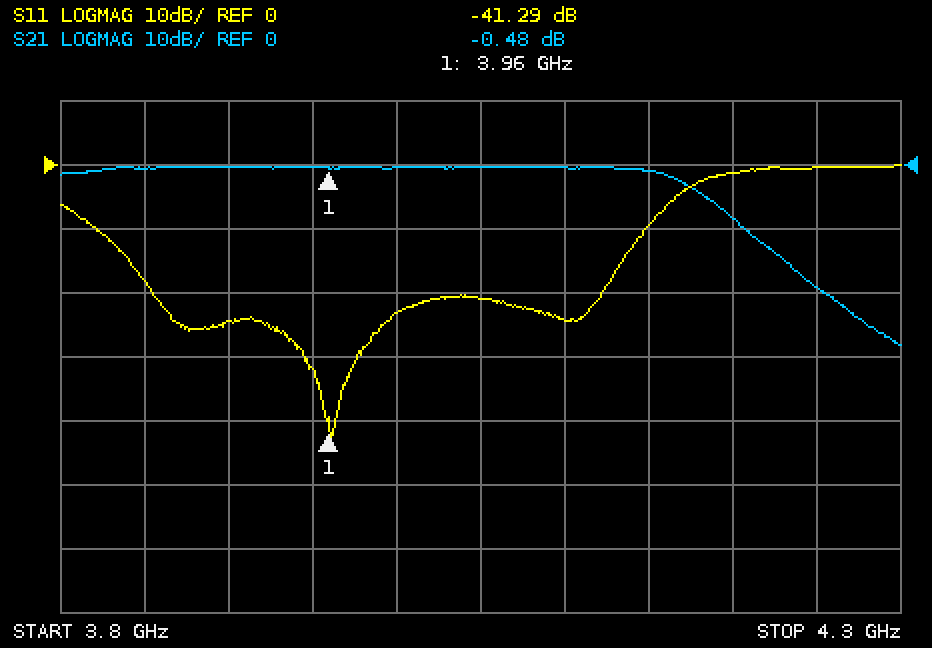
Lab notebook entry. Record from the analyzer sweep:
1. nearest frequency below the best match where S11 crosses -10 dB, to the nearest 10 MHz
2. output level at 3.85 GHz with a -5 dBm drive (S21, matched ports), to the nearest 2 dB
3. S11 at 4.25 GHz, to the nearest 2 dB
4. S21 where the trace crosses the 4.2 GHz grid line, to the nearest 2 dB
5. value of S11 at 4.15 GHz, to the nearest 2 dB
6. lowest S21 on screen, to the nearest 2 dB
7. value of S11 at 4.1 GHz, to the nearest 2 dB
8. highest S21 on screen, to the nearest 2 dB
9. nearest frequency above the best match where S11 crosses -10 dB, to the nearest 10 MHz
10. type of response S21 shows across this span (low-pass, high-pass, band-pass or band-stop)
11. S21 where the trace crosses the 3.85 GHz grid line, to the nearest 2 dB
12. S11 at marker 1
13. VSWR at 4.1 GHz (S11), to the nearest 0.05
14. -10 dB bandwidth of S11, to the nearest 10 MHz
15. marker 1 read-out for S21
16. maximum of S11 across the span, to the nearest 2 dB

3.82 GHz
-6 dBm
0 dB
-8 dB
-10 dB
-28 dB
-24 dB
0 dB
4.15 GHz
low-pass
0 dB
-41.29 dB
1.15
330 MHz
-0.48 dB
0 dB
